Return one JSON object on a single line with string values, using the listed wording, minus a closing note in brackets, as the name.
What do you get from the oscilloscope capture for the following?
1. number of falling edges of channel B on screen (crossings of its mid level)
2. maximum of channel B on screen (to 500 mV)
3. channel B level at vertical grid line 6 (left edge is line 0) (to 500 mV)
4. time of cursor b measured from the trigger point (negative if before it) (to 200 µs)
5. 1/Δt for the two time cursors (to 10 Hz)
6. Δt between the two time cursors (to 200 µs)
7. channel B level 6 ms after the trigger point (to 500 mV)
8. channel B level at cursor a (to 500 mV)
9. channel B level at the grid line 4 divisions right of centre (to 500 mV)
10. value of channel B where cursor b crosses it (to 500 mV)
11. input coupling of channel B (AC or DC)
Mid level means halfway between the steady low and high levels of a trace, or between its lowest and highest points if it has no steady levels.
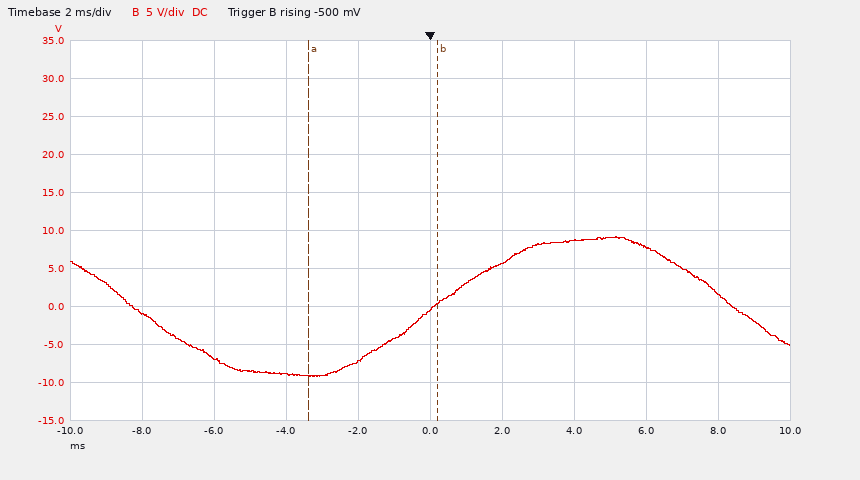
{"number of falling edges of channel B on screen": "2", "maximum of channel B on screen": "9.0 V", "channel B level at vertical grid line 6 (left edge is line 0)": "5.5 V", "time of cursor b measured from the trigger point (negative if before it)": "+200 µs", "1/Δt for the two time cursors": "280 Hz", "Δt between the two time cursors": "3.6 ms", "channel B level 6 ms after the trigger point": "8.0 V", "channel B level at cursor a": "-9.0 V", "channel B level at the grid line 4 divisions right of centre": "1.5 V", "value of channel B where cursor b crosses it": "500 mV", "input coupling of channel B": "DC"}
